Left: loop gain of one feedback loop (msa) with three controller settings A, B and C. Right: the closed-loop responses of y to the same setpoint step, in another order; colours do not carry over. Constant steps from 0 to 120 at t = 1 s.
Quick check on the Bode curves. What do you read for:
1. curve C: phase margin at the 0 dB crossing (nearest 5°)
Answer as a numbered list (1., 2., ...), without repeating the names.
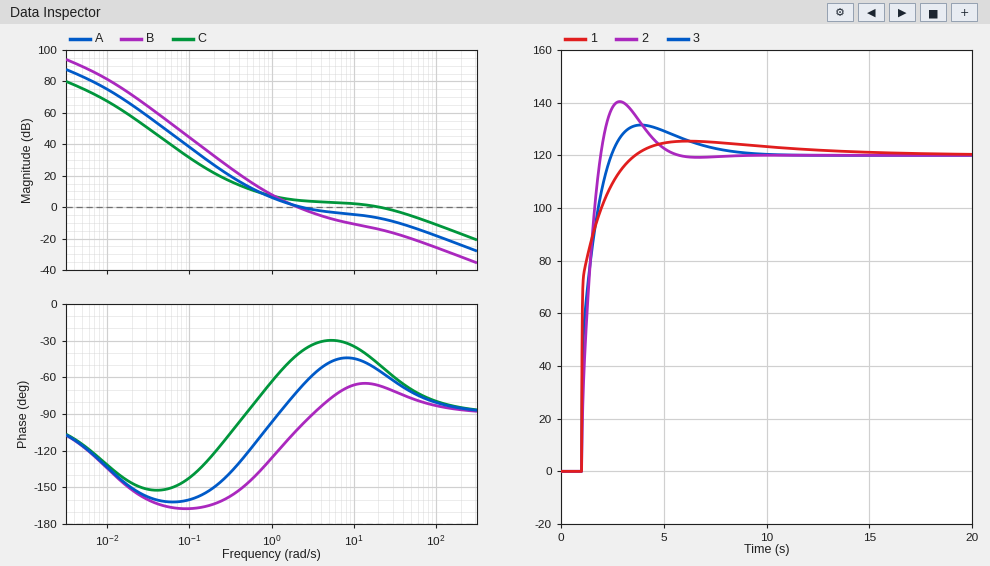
1. 130°
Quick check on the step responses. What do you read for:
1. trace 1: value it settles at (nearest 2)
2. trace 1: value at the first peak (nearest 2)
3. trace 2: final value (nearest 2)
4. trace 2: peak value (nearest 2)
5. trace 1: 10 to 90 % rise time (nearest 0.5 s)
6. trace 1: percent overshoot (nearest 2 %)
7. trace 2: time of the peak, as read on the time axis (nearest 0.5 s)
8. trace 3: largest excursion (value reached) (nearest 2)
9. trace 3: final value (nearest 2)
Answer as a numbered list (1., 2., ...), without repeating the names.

1. 120
2. 126
3. 120
4. 140
5. 1.5 s
6. 4 %
7. 3.0 s
8. 132
9. 120
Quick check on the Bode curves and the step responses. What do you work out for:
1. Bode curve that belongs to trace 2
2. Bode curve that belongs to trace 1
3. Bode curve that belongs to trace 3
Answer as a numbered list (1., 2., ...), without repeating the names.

1. B
2. C
3. A
